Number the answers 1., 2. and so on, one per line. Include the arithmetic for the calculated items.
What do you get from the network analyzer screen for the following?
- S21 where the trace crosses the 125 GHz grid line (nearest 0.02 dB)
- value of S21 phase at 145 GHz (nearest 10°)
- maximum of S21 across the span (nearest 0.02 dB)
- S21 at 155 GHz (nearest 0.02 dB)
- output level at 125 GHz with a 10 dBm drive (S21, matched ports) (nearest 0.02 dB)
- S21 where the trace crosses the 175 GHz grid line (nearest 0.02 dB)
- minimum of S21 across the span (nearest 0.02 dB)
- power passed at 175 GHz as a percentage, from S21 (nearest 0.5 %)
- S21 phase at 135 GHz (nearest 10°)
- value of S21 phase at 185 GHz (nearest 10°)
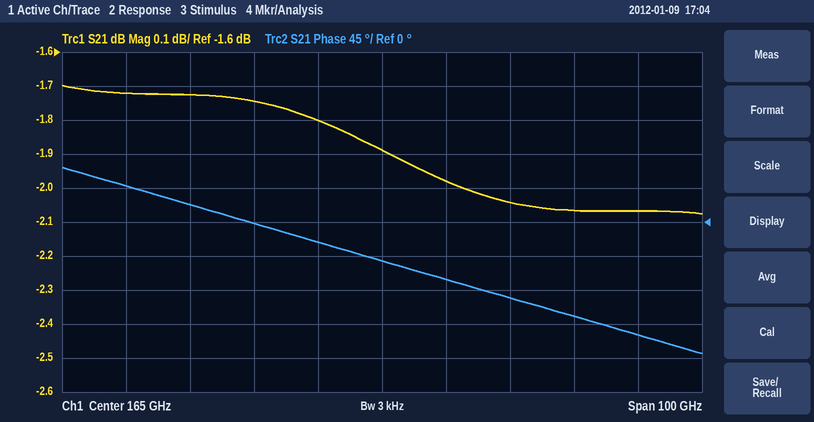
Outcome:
1. -1.72 dB
2. 0°
3. -1.70 dB
4. -1.80 dB
5. 10 dBm + (-1.72 dB) = 8.28 dBm
6. -1.98 dB
7. -2.08 dB
8. 10^(-1.98/10) ≈ 63.4 %, so 63.5 % to the nearest 0.5 %
9. 20°
10. -100°
